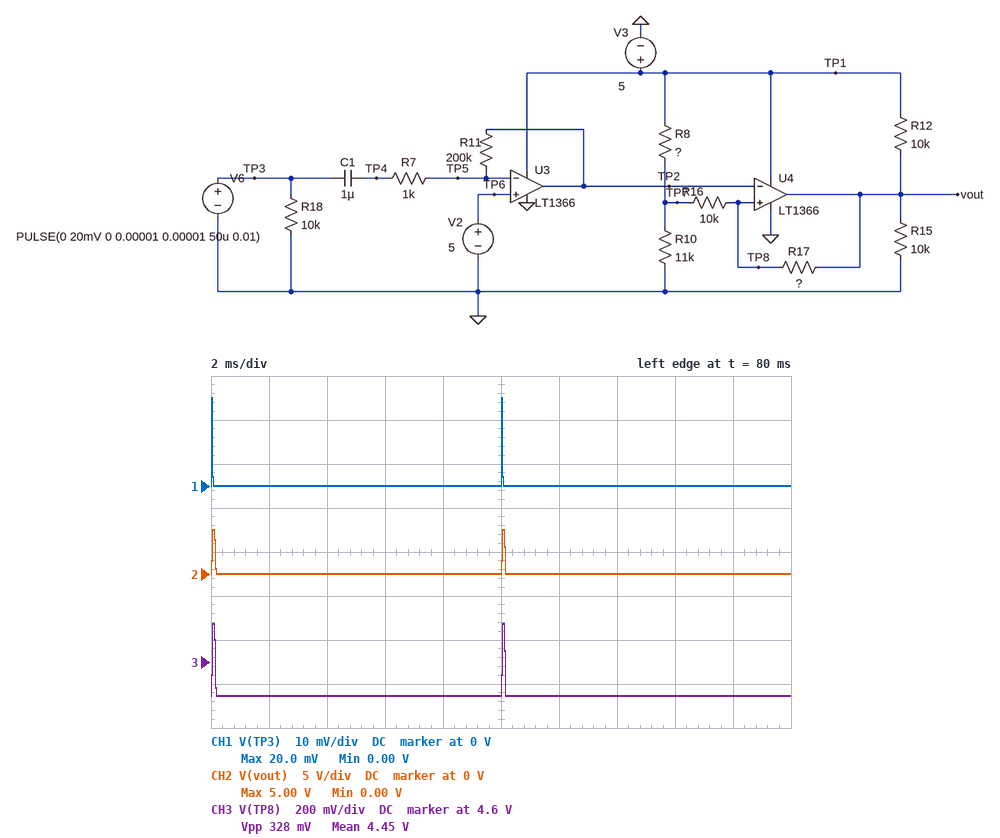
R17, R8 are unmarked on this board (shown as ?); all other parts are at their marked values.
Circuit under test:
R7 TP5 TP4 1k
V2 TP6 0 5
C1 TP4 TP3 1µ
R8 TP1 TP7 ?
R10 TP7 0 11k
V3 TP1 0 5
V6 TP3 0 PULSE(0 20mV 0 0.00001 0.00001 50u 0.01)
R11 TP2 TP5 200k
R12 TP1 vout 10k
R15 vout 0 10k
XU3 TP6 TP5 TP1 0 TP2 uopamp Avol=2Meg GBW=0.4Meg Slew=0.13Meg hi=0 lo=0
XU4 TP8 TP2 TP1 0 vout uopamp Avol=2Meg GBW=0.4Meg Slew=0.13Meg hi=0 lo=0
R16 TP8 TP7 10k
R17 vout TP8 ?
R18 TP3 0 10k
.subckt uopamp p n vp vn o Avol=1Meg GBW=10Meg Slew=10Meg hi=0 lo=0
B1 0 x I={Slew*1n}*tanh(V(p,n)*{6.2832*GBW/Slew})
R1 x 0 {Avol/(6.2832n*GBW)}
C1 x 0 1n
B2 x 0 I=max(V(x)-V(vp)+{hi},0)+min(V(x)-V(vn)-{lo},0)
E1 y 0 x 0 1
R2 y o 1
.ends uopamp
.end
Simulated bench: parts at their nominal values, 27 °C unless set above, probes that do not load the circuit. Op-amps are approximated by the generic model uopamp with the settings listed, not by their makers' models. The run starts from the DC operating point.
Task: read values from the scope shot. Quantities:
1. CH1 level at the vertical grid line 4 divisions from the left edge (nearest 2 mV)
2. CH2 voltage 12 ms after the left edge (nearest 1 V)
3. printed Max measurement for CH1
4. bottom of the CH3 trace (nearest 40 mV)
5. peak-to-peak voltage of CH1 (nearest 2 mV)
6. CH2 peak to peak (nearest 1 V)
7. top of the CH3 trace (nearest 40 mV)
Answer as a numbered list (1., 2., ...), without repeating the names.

1. 0 V
2. 0 V
3. 20.0 mV
4. 4.44 V
5. 20 mV
6. 5 V
7. 4.76 V
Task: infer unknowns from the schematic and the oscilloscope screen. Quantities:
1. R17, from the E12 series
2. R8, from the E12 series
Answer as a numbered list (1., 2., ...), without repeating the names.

1. 150 kΩ
2. 560 Ω
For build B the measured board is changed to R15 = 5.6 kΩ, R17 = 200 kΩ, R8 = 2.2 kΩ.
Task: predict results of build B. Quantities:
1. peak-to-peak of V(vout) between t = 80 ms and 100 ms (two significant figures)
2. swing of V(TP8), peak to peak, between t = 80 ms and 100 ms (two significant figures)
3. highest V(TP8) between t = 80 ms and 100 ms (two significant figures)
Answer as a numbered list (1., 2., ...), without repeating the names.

1. 5.0 V
2. 280 mV
3. 4.2 V
